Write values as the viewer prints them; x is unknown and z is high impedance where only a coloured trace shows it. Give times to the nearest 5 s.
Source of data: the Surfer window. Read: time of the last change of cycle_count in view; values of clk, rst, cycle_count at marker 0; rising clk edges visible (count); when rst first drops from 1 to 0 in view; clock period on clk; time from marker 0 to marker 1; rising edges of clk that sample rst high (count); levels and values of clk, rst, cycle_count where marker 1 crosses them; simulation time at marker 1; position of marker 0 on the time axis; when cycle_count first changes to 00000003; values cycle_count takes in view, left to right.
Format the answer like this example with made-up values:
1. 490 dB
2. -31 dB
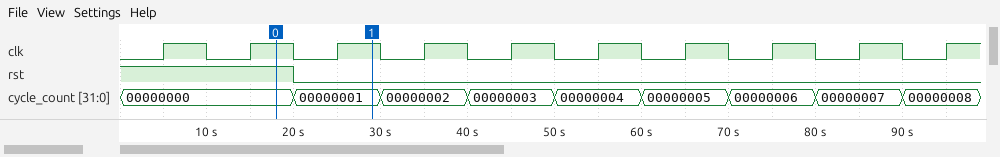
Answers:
1. 90 s
2. clk=1, rst=1, cycle_count=00000000
3. 10
4. 20 s
5. 10 s
6. 10 s
7. 2
8. clk=1, rst=0, cycle_count=00000001
9. 30 s
10. 20 s
11. 40 s
12. 00000000, 00000001, 00000002, 00000003, 00000004, 00000005, 00000006, 00000007, 00000008
